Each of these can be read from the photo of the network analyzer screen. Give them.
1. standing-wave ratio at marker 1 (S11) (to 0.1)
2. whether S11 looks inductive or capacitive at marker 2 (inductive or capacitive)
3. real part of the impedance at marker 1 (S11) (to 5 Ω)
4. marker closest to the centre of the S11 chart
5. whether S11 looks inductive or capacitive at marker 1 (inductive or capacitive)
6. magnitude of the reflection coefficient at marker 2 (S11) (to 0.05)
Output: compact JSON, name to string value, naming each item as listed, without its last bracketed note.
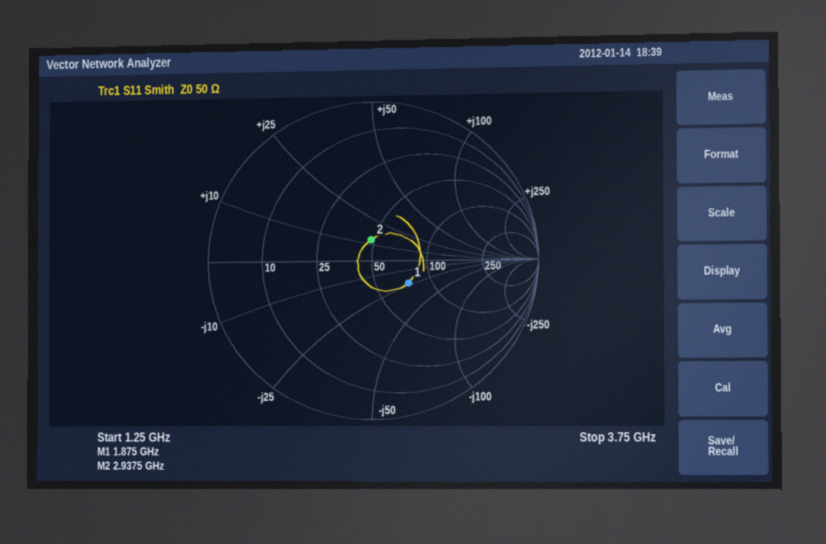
{"standing-wave ratio at marker 1 (S11)": "1.7", "whether S11 looks inductive or capacitive at marker 2": "inductive", "real part of the impedance at marker 1 (S11)": "75 Ω", "marker closest to the centre of the S11 chart": "marker 2", "whether S11 looks inductive or capacitive at marker 1": "capacitive", "magnitude of the reflection coefficient at marker 2 (S11)": "0.15"}
